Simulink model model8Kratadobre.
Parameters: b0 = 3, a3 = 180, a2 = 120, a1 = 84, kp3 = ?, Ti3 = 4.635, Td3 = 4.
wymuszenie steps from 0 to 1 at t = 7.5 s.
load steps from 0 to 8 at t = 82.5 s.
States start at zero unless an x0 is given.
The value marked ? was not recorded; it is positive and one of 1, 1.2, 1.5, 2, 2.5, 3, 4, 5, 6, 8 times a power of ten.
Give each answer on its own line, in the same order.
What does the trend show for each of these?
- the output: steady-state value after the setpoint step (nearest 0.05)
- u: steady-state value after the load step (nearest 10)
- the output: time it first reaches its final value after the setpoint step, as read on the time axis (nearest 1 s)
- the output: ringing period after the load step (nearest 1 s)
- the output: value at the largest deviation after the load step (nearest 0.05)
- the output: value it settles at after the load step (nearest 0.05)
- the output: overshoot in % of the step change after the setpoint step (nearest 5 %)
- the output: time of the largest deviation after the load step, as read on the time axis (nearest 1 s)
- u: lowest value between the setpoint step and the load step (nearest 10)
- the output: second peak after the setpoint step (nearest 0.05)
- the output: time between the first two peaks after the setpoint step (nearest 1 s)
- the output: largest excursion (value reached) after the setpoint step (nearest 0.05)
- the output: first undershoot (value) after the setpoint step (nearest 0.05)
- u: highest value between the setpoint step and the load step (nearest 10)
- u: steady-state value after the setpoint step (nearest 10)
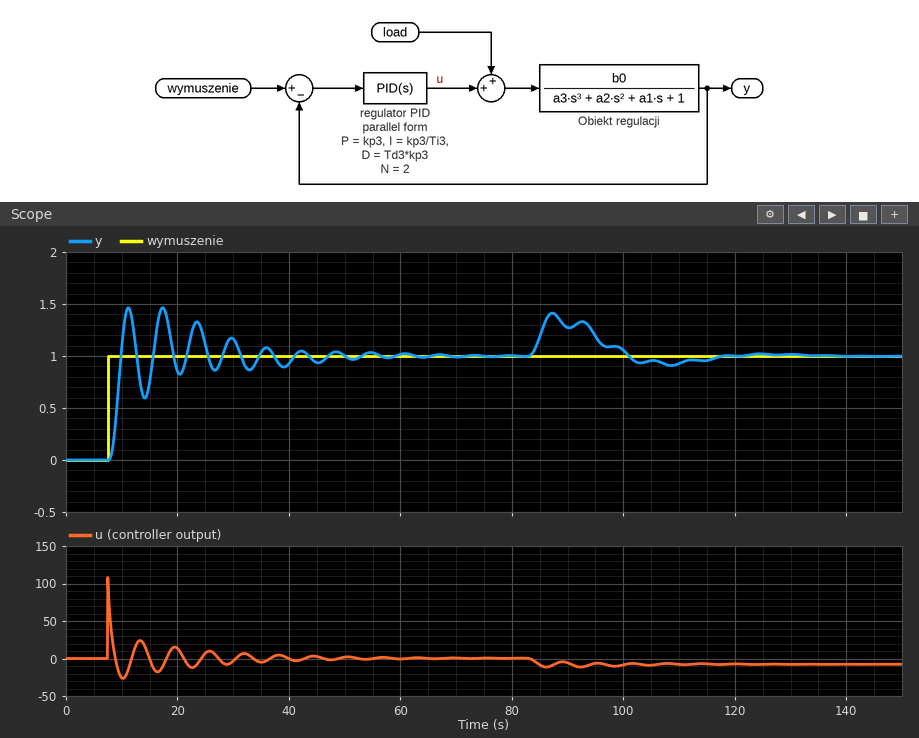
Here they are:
1.00
-10
10 s
5 s
1.40
1.00
45 %
87 s
-30
1.45
6 s
1.45
0.60
110
0
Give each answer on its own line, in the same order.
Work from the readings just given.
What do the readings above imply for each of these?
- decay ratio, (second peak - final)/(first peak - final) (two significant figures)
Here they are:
1.0
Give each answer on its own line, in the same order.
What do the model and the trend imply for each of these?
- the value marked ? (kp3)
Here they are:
12
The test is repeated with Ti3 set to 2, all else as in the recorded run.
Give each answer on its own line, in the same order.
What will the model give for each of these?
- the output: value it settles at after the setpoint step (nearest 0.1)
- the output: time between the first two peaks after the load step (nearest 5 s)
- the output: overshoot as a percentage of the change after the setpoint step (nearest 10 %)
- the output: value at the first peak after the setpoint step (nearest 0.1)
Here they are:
1.0
20 s
60 %
1.6
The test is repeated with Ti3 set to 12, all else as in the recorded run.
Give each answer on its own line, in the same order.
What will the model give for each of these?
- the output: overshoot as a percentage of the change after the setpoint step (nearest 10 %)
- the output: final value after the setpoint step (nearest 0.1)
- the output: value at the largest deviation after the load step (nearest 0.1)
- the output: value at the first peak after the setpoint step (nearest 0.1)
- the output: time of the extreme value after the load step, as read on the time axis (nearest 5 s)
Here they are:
40 %
1.0
1.5
1.4
95 s
